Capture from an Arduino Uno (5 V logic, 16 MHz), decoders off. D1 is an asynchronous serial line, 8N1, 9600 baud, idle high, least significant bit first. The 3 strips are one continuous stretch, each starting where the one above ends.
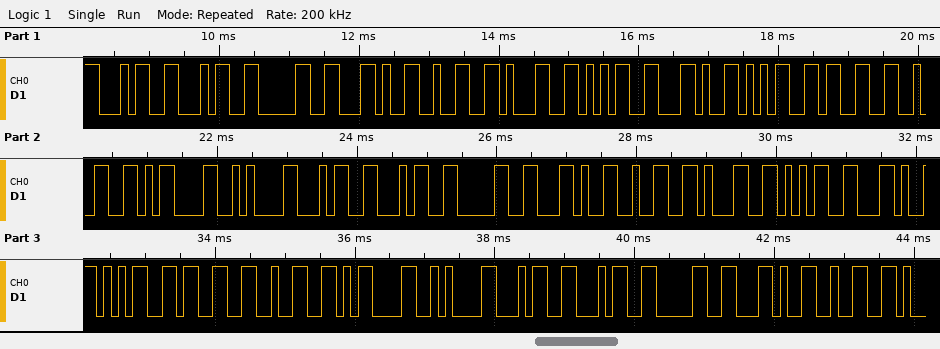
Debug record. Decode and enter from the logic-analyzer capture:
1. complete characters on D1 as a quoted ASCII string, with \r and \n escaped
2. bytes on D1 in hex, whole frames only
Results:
"440,215,532\r\n440,215,532\r\n440,2"
34 34 30 2C 32 31 35 2C 35 33 32 0D 0A 34 34 30 2C 32 31 35 2C 35 33 32 0D 0A 34 34 30 2C 32
